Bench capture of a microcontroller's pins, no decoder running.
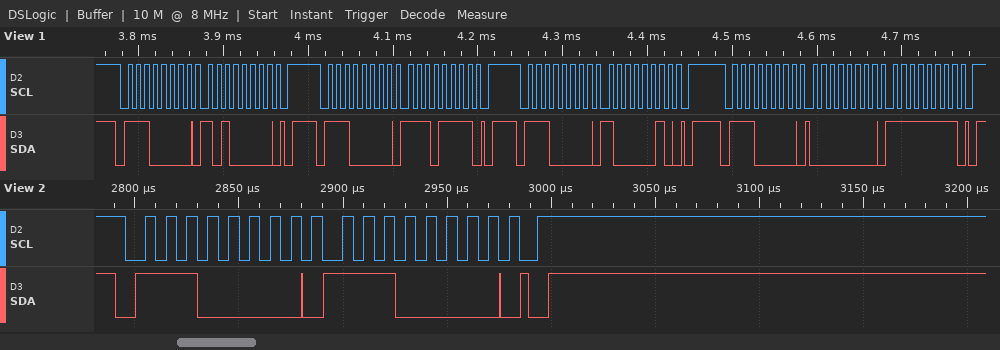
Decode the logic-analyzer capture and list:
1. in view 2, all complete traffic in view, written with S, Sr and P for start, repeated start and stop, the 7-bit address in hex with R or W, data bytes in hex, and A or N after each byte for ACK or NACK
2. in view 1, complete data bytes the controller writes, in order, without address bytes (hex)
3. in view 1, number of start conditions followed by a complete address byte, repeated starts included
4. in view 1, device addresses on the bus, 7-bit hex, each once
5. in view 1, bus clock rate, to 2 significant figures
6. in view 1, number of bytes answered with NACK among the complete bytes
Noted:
S 70W A E0 A P
A0 EF 82 00 FF
4
0x70
100 kHz
0
